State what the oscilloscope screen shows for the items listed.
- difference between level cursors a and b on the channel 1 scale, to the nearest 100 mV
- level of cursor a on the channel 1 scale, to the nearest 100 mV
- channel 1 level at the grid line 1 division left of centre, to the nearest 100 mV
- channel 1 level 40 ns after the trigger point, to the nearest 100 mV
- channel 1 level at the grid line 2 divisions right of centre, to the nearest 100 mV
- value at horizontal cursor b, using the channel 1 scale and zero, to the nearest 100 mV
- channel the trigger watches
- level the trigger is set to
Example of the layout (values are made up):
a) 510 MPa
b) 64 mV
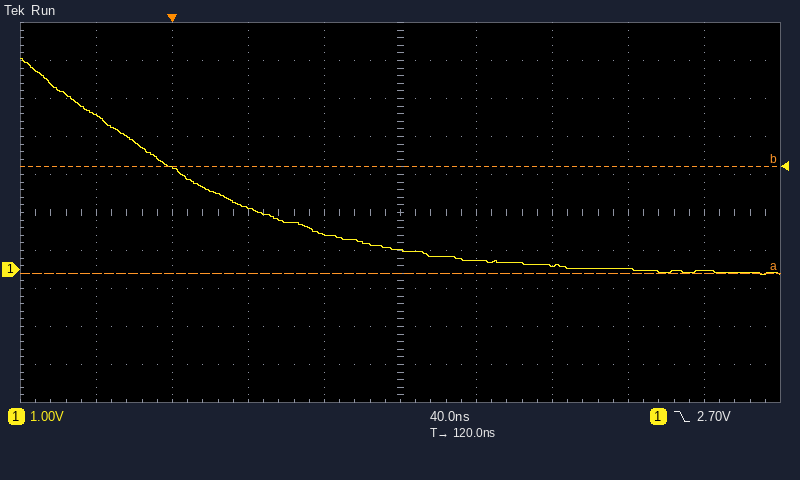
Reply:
a) 2.8 V
b) -100 mV
c) 900 mV
d) 1.6 V
e) 100 mV
f) 2.7 V
g) channel 1
h) 2.70 V
